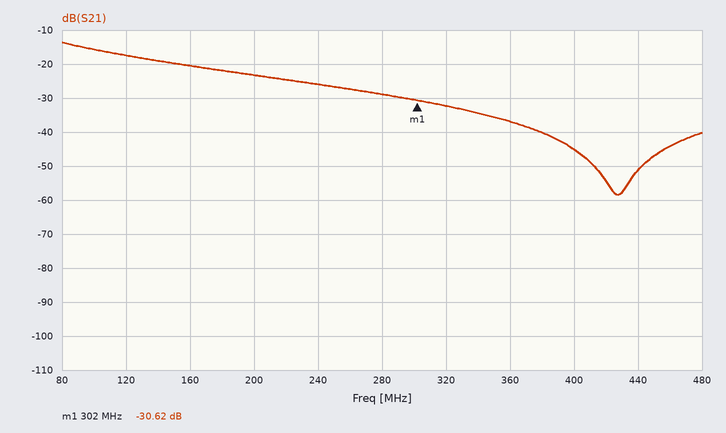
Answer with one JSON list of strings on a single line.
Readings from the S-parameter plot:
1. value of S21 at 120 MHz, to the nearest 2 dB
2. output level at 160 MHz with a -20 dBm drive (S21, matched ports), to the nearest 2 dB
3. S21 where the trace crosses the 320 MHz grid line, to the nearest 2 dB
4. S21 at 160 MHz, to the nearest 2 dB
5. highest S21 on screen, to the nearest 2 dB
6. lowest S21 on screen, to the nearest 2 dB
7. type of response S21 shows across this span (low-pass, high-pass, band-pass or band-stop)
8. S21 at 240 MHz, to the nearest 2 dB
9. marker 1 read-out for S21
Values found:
["-18 dB", "-40 dBm", "-32 dB", "-20 dB", "-14 dB", "-58 dB", "low-pass", "-26 dB", "-30.62 dB"]
